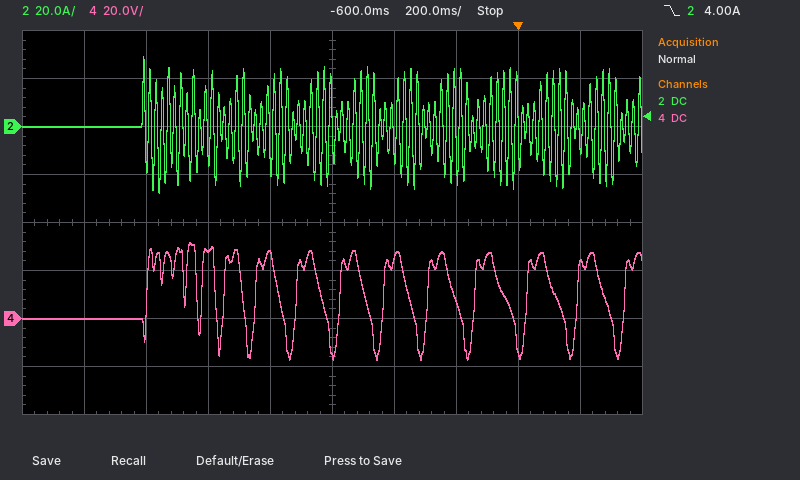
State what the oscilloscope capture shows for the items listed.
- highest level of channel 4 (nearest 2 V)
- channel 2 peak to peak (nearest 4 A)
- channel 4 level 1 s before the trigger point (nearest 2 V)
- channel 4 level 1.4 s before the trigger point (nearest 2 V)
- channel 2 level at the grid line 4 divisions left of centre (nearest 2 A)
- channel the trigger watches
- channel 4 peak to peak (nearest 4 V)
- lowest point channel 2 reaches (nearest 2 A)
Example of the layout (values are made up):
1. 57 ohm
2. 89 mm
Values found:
1. 32 V
2. 56 A
3. 28 V
4. 0 V
5. 0 A
6. channel 2
7. 48 V
8. -28 A
